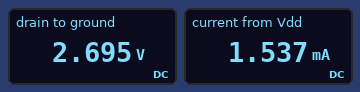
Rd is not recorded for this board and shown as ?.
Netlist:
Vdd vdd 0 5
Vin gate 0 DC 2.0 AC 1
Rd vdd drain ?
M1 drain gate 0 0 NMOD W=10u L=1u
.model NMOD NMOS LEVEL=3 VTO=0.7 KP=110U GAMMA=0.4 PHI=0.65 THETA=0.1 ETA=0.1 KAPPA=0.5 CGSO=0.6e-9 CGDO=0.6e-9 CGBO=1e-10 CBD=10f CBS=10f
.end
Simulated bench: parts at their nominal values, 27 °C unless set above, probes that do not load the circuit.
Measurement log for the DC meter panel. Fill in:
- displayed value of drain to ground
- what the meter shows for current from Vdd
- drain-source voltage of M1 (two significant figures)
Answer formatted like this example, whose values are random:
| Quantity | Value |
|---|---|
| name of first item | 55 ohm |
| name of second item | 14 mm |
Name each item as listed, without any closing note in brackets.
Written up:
| Quantity | Value |
|---|---|
| displayed value of drain to ground | 2.695 V |
| what the meter shows for current from Vdd | 1.537 mA |
| drain-source voltage of M1 | 2.7 V |
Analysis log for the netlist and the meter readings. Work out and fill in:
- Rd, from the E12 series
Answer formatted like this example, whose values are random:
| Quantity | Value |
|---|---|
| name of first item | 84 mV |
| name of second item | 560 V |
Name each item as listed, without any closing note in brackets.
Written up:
| Quantity | Value |
|---|---|
| Rd, from the E12 series | 1.5 kΩ |
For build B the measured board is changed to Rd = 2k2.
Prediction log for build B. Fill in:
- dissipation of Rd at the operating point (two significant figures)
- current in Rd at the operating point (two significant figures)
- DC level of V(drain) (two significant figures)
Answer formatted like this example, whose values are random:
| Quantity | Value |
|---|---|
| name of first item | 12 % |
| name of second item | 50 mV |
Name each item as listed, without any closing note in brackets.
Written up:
| Quantity | Value |
|---|---|
| dissipation of Rd at the operating point | 3.9 mW |
| current in Rd at the operating point | 1.3 mA |
| DC level of V(drain) | 2.1 V |
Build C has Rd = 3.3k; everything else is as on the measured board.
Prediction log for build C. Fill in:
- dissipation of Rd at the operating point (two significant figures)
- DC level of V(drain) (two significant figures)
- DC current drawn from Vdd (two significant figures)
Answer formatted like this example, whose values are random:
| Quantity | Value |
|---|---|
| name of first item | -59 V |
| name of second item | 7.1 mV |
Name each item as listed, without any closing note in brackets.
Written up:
| Quantity | Value |
|---|---|
| dissipation of Rd at the operating point | 4.0 mW |
| DC level of V(drain) | 1.4 V |
| DC current drawn from Vdd | 1.1 mA |
